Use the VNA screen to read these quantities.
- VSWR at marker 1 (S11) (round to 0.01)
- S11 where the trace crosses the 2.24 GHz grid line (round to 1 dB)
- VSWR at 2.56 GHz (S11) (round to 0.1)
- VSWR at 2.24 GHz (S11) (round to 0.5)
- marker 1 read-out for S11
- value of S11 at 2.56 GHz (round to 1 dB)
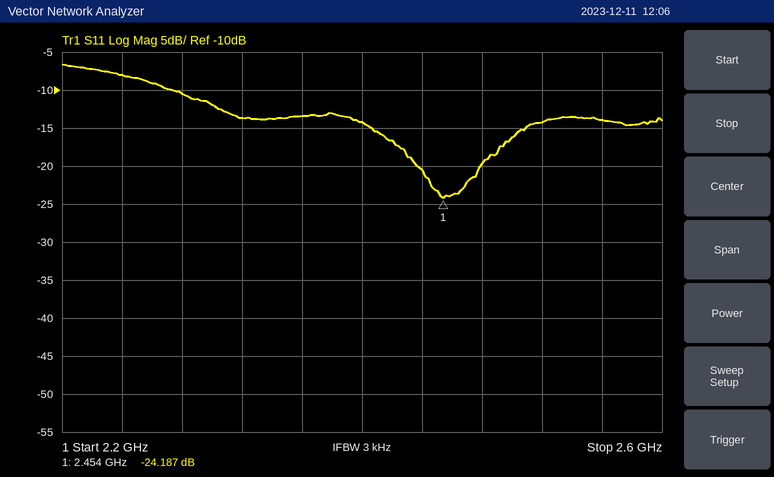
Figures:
1.13
-8 dB
1.5
2.5
-24.187 dB
-14 dB
